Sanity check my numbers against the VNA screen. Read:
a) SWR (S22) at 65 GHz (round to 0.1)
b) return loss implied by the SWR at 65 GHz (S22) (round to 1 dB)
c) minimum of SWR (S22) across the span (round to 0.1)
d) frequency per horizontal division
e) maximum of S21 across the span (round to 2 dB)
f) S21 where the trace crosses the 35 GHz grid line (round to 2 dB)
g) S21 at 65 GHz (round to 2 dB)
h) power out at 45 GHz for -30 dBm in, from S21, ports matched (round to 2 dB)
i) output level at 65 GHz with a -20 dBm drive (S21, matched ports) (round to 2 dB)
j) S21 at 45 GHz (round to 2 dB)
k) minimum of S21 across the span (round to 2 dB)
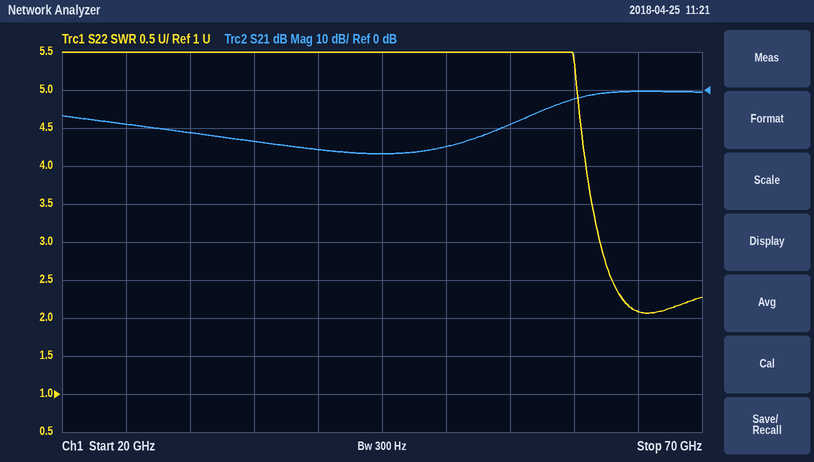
2.1
9 dB
2.1
5 GHz
0 dB
-14 dB
0 dB
-46 dBm
-20 dBm
-16 dB
-16 dB
